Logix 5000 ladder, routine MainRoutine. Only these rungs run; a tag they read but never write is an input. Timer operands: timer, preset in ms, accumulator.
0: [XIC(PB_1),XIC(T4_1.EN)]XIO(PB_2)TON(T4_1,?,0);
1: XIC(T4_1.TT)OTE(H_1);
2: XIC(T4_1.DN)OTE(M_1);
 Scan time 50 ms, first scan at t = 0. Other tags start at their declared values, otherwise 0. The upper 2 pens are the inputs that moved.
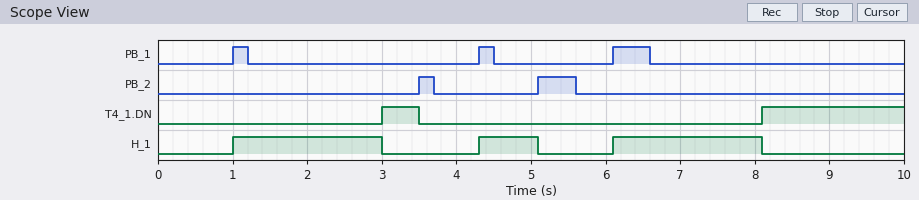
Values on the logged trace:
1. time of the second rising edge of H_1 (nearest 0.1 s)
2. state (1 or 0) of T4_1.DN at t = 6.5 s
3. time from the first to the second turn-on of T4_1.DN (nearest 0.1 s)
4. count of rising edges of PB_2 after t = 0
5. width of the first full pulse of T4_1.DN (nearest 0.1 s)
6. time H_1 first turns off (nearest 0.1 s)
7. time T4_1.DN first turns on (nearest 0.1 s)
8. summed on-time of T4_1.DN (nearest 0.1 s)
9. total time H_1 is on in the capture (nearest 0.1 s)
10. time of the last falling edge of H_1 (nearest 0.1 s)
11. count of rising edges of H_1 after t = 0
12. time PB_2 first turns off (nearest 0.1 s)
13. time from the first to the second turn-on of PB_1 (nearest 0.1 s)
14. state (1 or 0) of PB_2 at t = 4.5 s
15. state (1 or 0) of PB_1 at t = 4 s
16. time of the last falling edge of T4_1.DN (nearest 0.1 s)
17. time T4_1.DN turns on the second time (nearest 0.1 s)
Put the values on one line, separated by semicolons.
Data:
4.3 s; 0; 5.1 s; 2; 0.5 s; 3.0 s; 3.0 s; 2.4 s; 4.8 s; 8.1 s; 3; 3.7 s; 3.3 s; 0; 0; 3.5 s; 8.1 s
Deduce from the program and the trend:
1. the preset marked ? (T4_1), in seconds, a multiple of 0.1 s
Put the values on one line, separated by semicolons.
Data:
2.0 s
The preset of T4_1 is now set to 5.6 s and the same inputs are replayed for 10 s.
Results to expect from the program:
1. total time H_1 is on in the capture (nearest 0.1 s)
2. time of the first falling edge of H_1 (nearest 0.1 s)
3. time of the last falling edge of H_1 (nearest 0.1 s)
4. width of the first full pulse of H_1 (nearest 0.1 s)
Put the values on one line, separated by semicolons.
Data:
7.2 s; 3.5 s; 5.1 s; 2.5 s
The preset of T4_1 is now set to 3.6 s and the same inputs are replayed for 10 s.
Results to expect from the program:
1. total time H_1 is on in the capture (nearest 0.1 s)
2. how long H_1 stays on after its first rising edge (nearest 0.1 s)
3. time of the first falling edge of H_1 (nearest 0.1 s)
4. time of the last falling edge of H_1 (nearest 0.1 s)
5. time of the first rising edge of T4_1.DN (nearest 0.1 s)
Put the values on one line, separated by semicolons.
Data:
6.9 s; 2.5 s; 3.5 s; 9.7 s; 9.7 s
